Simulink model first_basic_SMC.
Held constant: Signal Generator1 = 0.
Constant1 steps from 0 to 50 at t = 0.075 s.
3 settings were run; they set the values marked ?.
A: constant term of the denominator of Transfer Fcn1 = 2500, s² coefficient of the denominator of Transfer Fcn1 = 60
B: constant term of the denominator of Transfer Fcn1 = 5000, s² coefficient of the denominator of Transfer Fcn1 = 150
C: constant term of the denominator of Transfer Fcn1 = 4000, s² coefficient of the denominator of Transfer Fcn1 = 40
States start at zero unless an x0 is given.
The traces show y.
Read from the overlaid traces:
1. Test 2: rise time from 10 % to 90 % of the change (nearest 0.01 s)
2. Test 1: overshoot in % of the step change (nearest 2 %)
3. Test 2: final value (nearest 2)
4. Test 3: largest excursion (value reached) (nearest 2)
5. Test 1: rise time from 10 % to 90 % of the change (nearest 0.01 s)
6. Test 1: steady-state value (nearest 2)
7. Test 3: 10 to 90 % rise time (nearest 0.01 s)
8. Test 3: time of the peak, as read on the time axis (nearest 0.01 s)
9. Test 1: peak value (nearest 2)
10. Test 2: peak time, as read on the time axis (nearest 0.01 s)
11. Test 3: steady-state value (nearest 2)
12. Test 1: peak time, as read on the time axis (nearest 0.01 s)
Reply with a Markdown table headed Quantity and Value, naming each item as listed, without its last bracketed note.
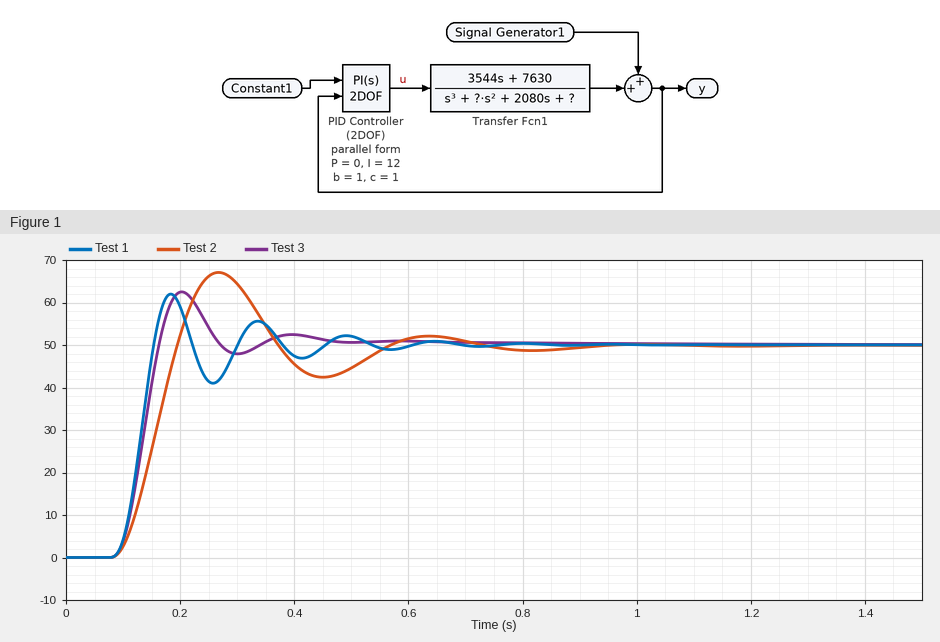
| Quantity | Value |
|---|---|
| Test 2: rise time from 10 % to 90 % of the change | 0.08 s |
| Test 1: overshoot in % of the step change | 24 % |
| Test 2: final value | 50 |
| Test 3: largest excursion (value reached) | 62 |
| Test 1: rise time from 10 % to 90 % of the change | 0.05 s |
| Test 1: steady-state value | 50 |
| Test 3: 10 to 90 % rise time | 0.05 s |
| Test 3: time of the peak, as read on the time axis | 0.20 s |
| Test 1: peak value | 62 |
| Test 2: peak time, as read on the time axis | 0.27 s |
| Test 3: steady-state value | 50 |
| Test 1: peak time, as read on the time axis | 0.18 s |
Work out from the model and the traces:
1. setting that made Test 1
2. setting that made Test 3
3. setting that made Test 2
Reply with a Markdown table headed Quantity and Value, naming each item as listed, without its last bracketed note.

| Quantity | Value |
|---|---|
| setting that made Test 1 | C |
| setting that made Test 3 | A |
| setting that made Test 2 | B |
